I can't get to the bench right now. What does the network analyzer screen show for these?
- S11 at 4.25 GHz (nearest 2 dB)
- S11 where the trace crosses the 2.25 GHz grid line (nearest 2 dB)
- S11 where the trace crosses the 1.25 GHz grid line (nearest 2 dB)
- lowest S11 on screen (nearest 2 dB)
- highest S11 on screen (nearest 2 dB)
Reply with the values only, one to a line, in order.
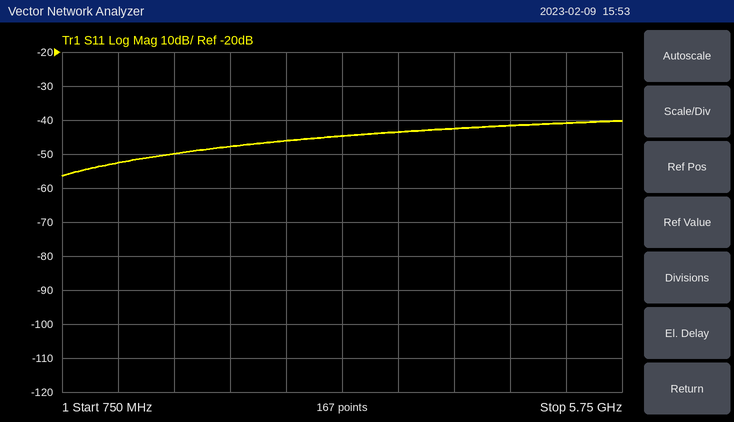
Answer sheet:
-42 dB
-48 dB
-52 dB
-56 dB
-40 dB
